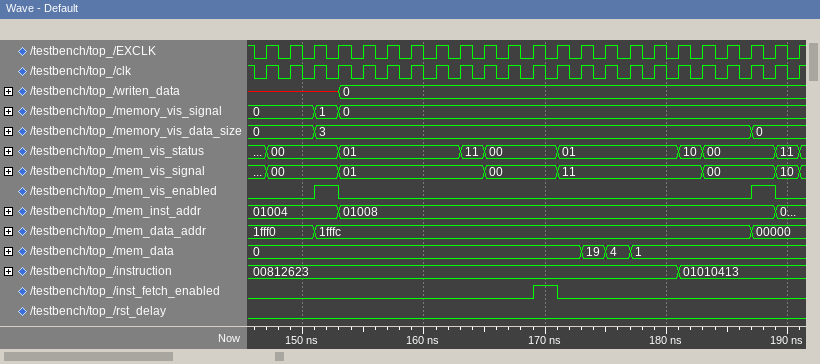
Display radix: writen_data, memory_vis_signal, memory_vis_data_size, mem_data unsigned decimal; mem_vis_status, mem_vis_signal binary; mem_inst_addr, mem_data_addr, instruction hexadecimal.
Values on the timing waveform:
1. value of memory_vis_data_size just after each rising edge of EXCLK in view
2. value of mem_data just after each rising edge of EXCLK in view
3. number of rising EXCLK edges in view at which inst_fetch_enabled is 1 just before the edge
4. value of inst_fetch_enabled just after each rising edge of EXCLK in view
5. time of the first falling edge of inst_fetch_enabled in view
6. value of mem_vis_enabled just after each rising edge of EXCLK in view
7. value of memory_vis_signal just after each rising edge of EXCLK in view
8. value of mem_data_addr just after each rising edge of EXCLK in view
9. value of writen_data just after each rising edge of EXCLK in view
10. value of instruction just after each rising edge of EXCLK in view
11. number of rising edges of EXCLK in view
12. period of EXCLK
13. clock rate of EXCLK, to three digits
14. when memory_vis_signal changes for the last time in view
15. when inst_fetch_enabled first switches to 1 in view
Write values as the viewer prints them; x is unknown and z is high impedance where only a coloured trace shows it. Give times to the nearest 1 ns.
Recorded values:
0, 0, 3, 3, 3, 3, 3, 3, 3, 3, 3, 3, 3, 3, 3, 3, 3, 3, 3, 3, 0, 0, 0
0, 0, 0, 0, 0, 0, 0, 0, 0, 0, 0, 0, 0, 19, 4, 1, 1, 1, 1, 1, 1, 1, 1
1
0 0 0 0 0 0 0 0 0 0 0 1 0 0 0 0 0 0 0 0 0 0 0
171 ns
0 0 1 0 0 0 0 0 0 0 0 0 0 0 0 0 0 0 0 0 1 0 0
0, 0, 1, 0, 0, 0, 0, 0, 0, 0, 0, 0, 0, 0, 0, 0, 0, 0, 0, 0, 0, 0, 0
1fff0, 1fff0, 1fffc, 1fffc, 1fffc, 1fffc, 1fffc, 1fffc, 1fffc, 1fffc, 1fffc, 1fffc, 1fffc, 1fffc, 1fffc, 1fffc, 1fffc, 1fffc, 1fffc, 1fffc, 00000, 00000, 00000
x, x, x, 0, 0, 0, 0, 0, 0, 0, 0, 0, 0, 0, 0, 0, 0, 0, 0, 0, 0, 0, 0
00812623, 00812623, 00812623, 00812623, 00812623, 00812623, 00812623, 00812623, 00812623, 00812623, 00812623, 00812623, 00812623, 00812623, 00812623, 00812623, 00812623, 01010413, 01010413, 01010413, 01010413, 01010413, 01010413
23
2 ns
500 MHz
153 ns
169 ns
